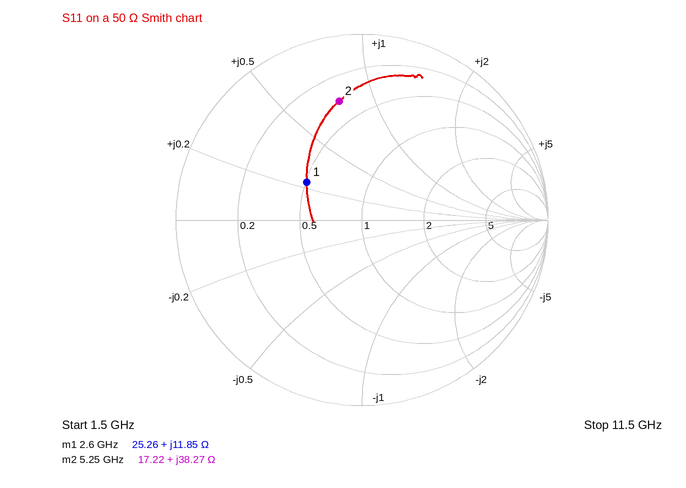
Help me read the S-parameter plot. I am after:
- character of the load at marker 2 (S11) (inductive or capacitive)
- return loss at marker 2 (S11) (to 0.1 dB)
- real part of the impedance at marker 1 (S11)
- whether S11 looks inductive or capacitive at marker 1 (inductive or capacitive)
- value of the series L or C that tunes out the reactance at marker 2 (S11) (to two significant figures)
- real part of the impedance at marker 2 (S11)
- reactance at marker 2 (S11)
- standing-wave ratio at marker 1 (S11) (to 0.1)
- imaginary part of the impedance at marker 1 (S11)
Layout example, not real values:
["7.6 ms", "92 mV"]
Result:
["inductive", "3.7 dB", "25.26 Ω", "inductive", "790 fF", "17.22 Ω", "+38.27 Ω", "2.1", "+11.85 Ω"]
